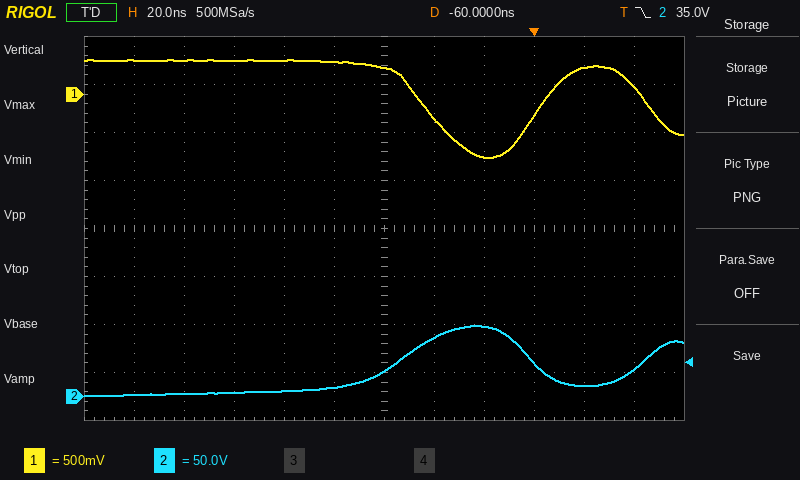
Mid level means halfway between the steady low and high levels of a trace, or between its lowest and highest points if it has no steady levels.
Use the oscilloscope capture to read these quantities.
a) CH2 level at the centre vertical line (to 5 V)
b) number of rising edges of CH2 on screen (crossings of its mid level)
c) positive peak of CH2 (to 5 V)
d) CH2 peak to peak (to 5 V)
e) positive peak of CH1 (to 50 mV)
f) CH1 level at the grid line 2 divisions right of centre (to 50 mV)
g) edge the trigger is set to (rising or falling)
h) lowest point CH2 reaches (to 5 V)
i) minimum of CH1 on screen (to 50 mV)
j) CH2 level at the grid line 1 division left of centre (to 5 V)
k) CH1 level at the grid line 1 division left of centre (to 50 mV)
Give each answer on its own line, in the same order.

25 V
2
75 V
75 V
350 mV
-650 mV
falling
0 V
-650 mV
10 V
350 mV
